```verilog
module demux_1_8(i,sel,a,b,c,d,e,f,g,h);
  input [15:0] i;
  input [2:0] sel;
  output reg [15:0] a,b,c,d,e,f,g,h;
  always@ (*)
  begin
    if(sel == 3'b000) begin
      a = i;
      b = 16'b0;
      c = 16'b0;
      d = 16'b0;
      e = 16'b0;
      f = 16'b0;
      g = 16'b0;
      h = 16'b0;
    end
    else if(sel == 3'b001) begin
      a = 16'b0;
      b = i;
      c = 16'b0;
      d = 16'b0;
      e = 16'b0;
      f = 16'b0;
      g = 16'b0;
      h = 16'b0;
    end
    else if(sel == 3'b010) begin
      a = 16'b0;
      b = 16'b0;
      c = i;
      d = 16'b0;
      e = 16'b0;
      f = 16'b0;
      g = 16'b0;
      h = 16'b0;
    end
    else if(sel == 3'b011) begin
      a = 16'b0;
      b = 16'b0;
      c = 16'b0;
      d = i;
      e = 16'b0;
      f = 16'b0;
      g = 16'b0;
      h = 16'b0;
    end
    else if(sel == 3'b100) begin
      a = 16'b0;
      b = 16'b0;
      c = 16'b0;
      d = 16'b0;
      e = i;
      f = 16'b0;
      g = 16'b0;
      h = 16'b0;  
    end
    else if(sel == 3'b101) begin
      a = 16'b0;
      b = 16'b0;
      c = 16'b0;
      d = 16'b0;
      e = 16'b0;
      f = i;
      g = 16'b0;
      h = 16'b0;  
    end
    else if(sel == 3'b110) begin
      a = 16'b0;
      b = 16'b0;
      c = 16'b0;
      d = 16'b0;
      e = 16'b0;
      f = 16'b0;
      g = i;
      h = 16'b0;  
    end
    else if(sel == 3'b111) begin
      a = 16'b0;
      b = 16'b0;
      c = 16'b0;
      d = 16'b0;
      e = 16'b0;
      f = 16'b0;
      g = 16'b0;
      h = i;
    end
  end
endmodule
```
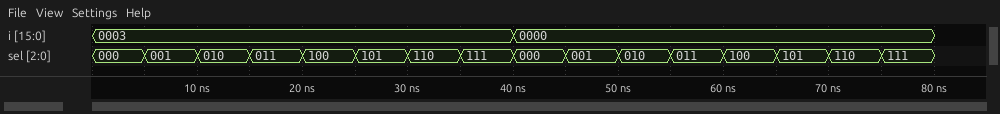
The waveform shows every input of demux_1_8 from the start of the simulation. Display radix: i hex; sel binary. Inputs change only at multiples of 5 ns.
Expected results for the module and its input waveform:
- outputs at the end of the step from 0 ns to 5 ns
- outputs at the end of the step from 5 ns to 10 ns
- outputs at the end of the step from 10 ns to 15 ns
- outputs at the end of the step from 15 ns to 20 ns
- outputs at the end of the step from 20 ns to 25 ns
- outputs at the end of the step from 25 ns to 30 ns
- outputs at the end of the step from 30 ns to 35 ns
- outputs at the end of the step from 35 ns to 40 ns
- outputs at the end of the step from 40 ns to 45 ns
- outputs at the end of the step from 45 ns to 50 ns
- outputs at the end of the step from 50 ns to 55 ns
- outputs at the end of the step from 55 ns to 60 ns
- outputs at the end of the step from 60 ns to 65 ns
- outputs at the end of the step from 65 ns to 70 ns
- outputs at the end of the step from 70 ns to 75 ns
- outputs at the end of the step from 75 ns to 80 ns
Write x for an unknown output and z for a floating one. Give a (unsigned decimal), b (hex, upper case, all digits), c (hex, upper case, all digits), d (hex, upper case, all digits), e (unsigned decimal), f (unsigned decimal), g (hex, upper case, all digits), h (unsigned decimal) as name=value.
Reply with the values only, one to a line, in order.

a=3, b=0000, c=0000, d=0000, e=0, f=0, g=0000, h=0
a=0, b=0003, c=0000, d=0000, e=0, f=0, g=0000, h=0
a=0, b=0000, c=0003, d=0000, e=0, f=0, g=0000, h=0
a=0, b=0000, c=0000, d=0003, e=0, f=0, g=0000, h=0
a=0, b=0000, c=0000, d=0000, e=3, f=0, g=0000, h=0
a=0, b=0000, c=0000, d=0000, e=0, f=3, g=0000, h=0
a=0, b=0000, c=0000, d=0000, e=0, f=0, g=0003, h=0
a=0, b=0000, c=0000, d=0000, e=0, f=0, g=0000, h=3
a=0, b=0000, c=0000, d=0000, e=0, f=0, g=0000, h=0
a=0, b=0000, c=0000, d=0000, e=0, f=0, g=0000, h=0
a=0, b=0000, c=0000, d=0000, e=0, f=0, g=0000, h=0
a=0, b=0000, c=0000, d=0000, e=0, f=0, g=0000, h=0
a=0, b=0000, c=0000, d=0000, e=0, f=0, g=0000, h=0
a=0, b=0000, c=0000, d=0000, e=0, f=0, g=0000, h=0
a=0, b=0000, c=0000, d=0000, e=0, f=0, g=0000, h=0
a=0, b=0000, c=0000, d=0000, e=0, f=0, g=0000, h=0
